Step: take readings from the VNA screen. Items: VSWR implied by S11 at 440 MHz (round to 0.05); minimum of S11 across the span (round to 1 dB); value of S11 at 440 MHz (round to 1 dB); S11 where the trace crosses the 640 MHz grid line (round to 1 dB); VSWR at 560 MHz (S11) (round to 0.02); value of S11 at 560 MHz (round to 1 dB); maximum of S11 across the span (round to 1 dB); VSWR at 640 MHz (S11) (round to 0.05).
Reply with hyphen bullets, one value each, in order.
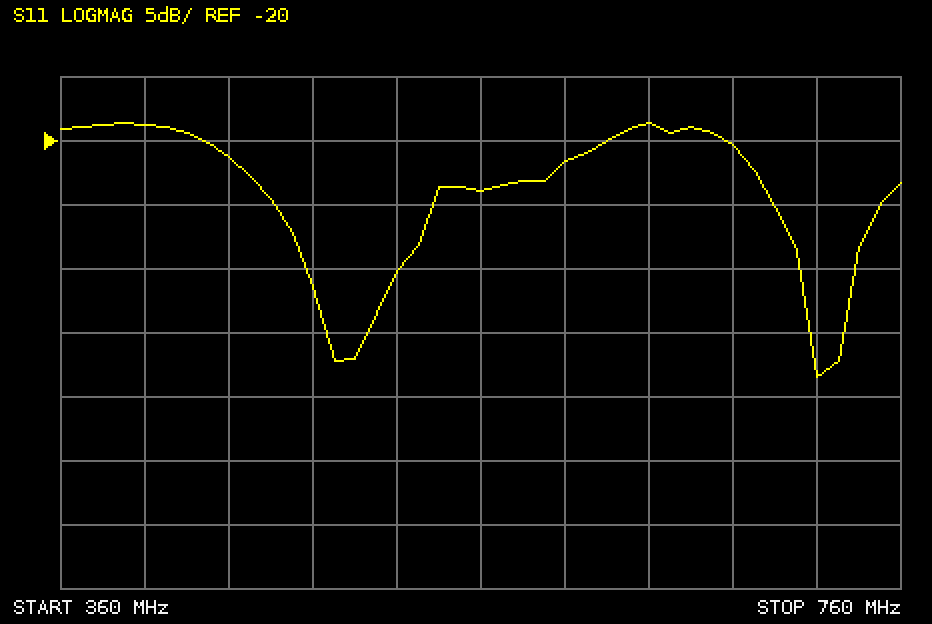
- 1.20
- -38 dB
- -21 dB
- -19 dB
- 1.14
- -24 dB
- -19 dB
- 1.25
